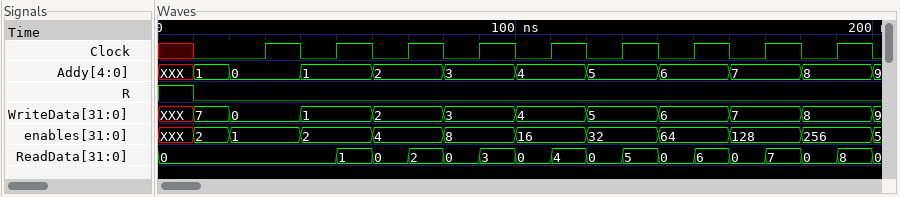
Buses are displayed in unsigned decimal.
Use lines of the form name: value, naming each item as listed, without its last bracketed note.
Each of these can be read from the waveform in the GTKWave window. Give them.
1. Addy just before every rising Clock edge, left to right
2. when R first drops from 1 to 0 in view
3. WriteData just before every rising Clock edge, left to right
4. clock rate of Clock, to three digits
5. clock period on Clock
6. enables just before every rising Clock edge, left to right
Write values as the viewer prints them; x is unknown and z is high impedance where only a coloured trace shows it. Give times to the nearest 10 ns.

Addy just before every rising Clock edge, left to right: 0, 1, 2, 3, 4, 5, 6, 7, 8
when R first drops from 1 to 0 in view: 10 ns
WriteData just before every rising Clock edge, left to right: 0, 1, 2, 3, 4, 5, 6, 7, 8
clock rate of Clock, to three digits: 50.0 MHz
clock period on Clock: 20 ns
enables just before every rising Clock edge, left to right: 1, 2, 4, 8, 16, 32, 64, 128, 256
